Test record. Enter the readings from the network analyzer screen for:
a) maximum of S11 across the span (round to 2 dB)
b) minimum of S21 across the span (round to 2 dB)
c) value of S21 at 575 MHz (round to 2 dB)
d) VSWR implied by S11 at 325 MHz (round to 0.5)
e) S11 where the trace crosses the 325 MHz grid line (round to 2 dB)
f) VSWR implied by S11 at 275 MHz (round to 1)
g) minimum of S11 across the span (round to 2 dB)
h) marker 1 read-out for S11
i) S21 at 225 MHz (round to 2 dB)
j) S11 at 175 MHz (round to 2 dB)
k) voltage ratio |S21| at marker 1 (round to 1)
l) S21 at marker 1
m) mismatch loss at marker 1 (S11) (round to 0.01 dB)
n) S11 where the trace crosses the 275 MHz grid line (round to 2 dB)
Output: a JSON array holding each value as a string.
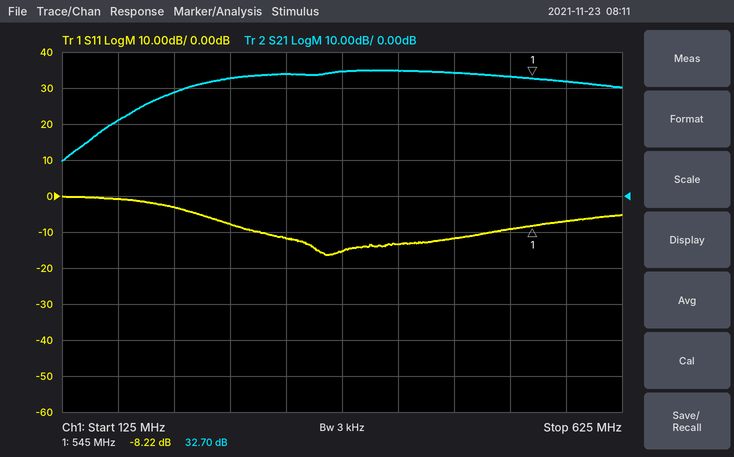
["0 dB", "10 dB", "32 dB", "1.5", "-12 dB", "2", "-16 dB", "-8.22 dB", "28 dB", "0 dB", "43", "32.70 dB", "0.71 dB", "-8 dB"]
